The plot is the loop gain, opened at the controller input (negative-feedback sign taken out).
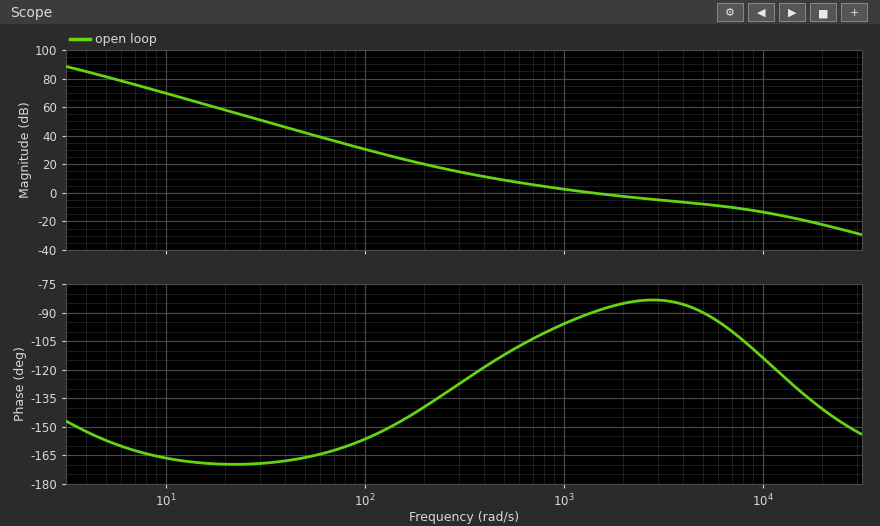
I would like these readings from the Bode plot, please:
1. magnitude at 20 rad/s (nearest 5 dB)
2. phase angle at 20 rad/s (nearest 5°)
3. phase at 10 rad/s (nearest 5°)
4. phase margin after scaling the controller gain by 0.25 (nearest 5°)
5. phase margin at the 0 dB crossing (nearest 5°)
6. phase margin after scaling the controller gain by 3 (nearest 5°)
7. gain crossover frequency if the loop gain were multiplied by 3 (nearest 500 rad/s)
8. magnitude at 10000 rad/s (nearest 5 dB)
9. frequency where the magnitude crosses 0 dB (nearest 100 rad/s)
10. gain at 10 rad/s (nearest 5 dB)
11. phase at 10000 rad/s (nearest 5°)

60 dB
-170°
-165°
60°
90°
85°
6500 rad/s
-15 dB
1400 rad/s
70 dB
-115°
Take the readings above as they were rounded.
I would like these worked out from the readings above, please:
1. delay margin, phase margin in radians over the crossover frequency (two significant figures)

0.0011 s
